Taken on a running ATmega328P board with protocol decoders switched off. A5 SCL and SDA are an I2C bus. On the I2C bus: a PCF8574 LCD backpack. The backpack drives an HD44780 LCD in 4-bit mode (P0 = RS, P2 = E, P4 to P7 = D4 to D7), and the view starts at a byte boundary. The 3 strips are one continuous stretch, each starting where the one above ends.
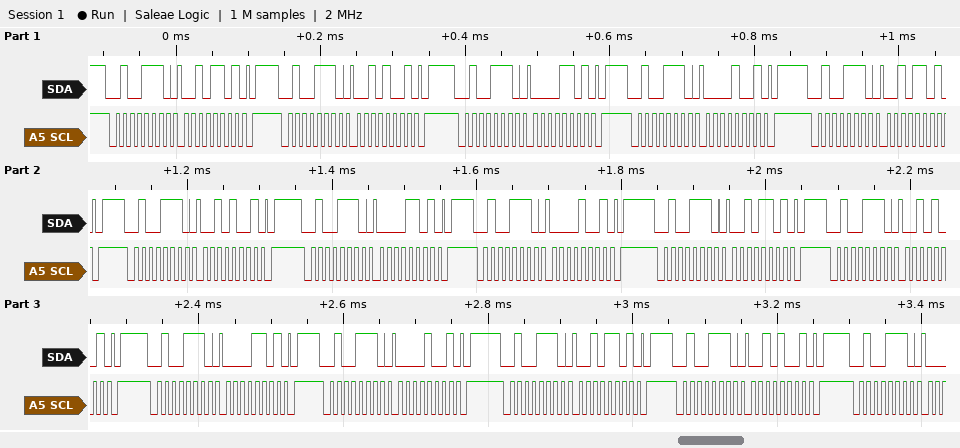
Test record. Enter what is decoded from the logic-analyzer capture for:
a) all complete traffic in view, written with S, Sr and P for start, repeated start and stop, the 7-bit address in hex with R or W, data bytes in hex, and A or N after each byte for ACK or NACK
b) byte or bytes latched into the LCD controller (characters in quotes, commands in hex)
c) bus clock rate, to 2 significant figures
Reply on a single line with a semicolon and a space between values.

S 27W A 2D A P S 27W A 29 A P S 27W A 0D A P S 27W A 09 A P S 27W A 2D A P S 27W A 29 A P S 27W A 0D A P S 27W A 09 A P S 27W A 2D A P S 27W A 29 A P S 27W A 0D A P S 27W A 09 A P S 27W A 2D A P S 27W A 29 A P S 27W A; ' ' ' ' ' '; 100 kHz
